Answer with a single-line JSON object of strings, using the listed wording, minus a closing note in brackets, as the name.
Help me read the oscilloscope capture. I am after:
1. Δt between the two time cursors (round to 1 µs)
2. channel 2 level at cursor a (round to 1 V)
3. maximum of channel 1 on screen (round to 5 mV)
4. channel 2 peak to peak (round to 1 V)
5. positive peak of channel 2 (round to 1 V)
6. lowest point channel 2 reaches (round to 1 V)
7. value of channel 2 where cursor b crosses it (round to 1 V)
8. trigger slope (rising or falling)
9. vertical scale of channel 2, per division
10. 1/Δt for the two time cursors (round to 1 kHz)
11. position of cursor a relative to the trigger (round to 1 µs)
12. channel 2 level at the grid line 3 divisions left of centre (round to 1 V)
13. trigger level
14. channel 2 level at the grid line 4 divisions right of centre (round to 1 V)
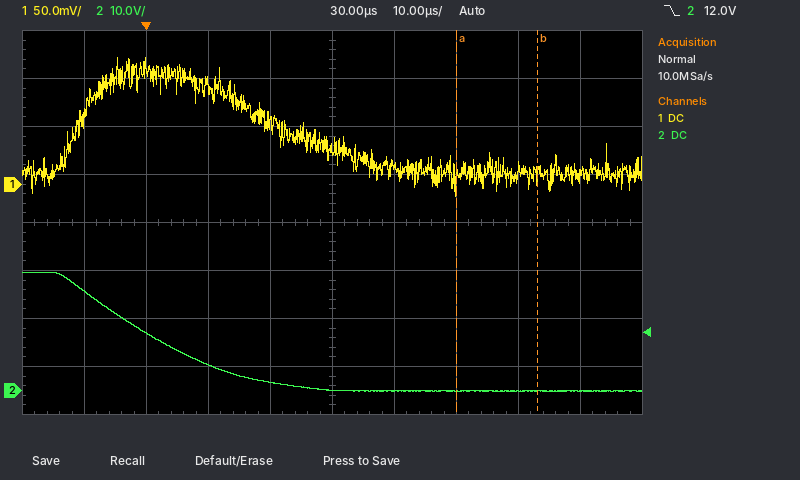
{"Δt between the two time cursors": "13 µs", "channel 2 level at cursor a": "0 V", "maximum of channel 1 on screen": "130 mV", "channel 2 peak to peak": "25 V", "positive peak of channel 2": "25 V", "lowest point channel 2 reaches": "0 V", "value of channel 2 where cursor b crosses it": "0 V", "trigger slope": "falling", "vertical scale of channel 2, per division": "10 V", "1/Δt for the two time cursors": "77 kHz", "position of cursor a relative to the trigger": "+50 µs", "channel 2 level at the grid line 3 divisions left of centre": "12 V", "trigger level": "12.0 V", "channel 2 level at the grid line 4 divisions right of centre": "0 V"}
